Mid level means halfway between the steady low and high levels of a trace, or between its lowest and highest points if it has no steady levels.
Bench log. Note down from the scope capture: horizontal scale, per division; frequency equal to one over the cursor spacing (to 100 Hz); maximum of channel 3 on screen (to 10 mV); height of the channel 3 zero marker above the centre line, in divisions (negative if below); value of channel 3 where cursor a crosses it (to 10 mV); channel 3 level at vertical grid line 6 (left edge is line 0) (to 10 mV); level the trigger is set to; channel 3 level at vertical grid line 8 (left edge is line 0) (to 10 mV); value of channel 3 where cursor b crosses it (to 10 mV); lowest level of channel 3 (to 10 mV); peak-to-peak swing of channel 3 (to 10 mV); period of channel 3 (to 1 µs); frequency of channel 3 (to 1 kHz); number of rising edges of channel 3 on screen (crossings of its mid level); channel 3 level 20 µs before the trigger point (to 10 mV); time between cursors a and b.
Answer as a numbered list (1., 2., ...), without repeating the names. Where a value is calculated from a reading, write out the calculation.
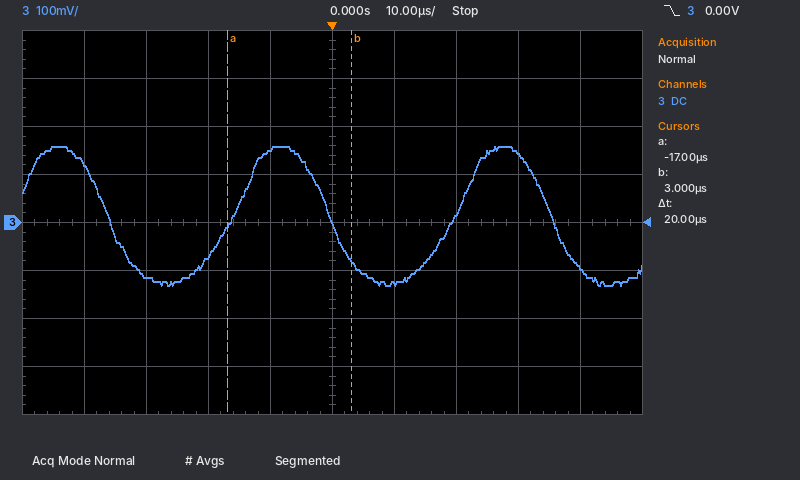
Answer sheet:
1. 10 µs
2. 1 / 20 µs ≈ 50.0 kHz
3. 160 mV
4. 0.0 div
5. -10 mV
6. -130 mV
7. 0.00 V
8. 140 mV
9. -80 mV
10. -130 mV
11. 160 mV − (-130 mV) = 290 mV
12. 36 µs
13. 1 / 36 µs ≈ 28 kHz
14. 2
15. -70 mV
16. 20 µs
